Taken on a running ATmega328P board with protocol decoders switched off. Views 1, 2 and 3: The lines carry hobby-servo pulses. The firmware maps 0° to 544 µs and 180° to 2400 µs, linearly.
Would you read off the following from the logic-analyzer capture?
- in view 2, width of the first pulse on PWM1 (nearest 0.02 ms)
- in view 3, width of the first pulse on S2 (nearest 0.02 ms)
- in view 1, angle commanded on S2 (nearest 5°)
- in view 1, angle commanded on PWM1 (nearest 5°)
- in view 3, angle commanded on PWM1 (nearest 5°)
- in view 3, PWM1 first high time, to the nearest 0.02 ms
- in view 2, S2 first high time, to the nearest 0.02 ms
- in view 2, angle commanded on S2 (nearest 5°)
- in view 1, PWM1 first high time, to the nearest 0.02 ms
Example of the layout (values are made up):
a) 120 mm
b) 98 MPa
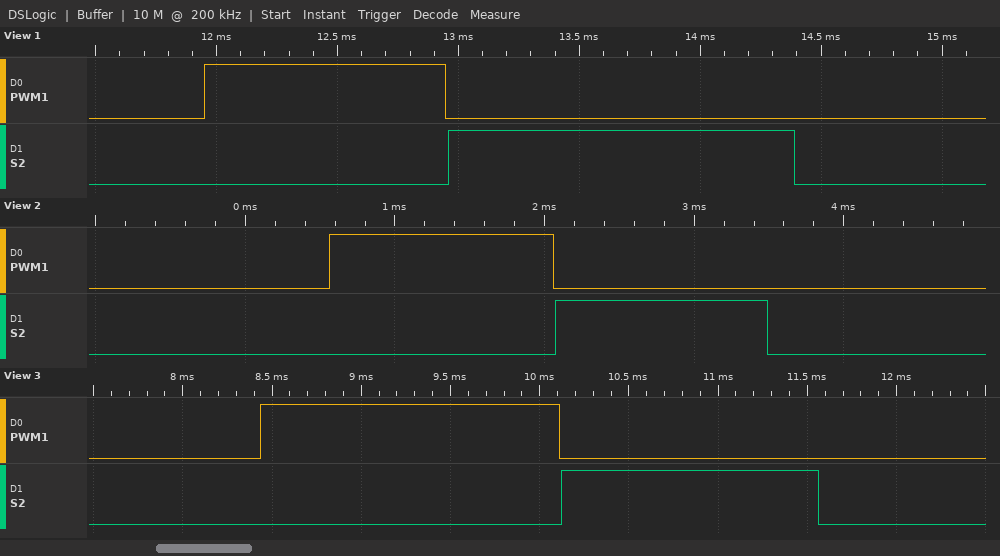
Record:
a) 1.50 ms
b) 1.44 ms
c) 85°
d) 45°
e) 110°
f) 1.68 ms
g) 1.42 ms
h) 85°
i) 1.00 ms
